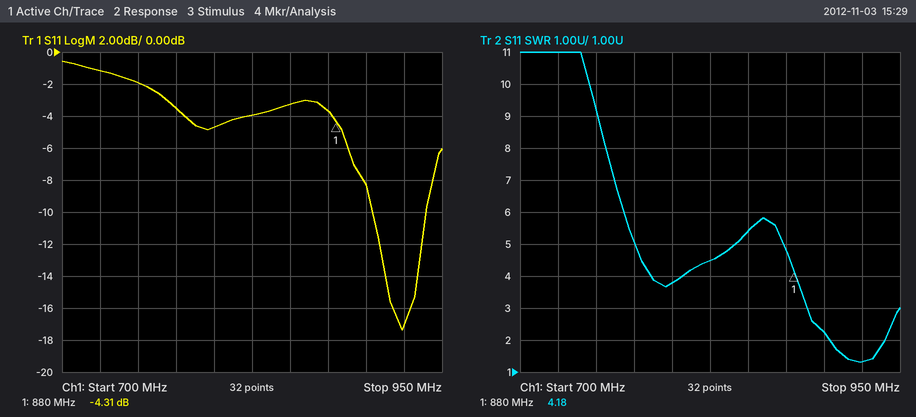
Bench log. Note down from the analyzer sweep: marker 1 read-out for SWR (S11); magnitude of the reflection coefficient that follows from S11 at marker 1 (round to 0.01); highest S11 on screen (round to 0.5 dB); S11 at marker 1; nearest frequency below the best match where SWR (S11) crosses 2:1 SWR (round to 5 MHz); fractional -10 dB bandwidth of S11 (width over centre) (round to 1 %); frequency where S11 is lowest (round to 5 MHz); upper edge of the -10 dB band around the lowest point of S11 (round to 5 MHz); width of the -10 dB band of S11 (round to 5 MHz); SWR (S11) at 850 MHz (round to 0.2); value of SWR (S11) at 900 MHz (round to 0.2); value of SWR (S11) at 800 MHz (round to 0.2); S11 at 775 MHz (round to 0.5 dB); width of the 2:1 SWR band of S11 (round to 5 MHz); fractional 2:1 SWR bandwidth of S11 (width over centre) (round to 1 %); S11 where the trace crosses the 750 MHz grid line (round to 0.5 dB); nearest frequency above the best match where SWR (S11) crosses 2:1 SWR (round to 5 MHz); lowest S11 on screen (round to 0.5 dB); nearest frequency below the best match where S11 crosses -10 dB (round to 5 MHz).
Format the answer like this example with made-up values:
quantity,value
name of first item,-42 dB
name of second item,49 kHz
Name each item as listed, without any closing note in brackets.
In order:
quantity,value
marker 1 read-out for SWR,4.18
magnitude of the reflection coefficient that follows from S11 at marker 1,0.61
highest S11 on screen,-0.5 dB
S11 at marker 1,-4.31 dB
nearest frequency below the best match where SWR (S11) crosses 2:1 SWR,905 MHz
fractional -10 dB bandwidth of S11 (width over centre),4 %
frequency where S11 is lowest,925 MHz
upper edge of the -10 dB band around the lowest point of S11,940 MHz
width of the -10 dB band of S11,35 MHz
SWR (S11) at 850 MHz,5.4
value of SWR (S11) at 900 MHz,2.2
value of SWR (S11) at 800 MHz,3.8
S11 at 775 MHz,-3.5 dB
width of the 2:1 SWR band of S11,35 MHz
fractional 2:1 SWR bandwidth of S11 (width over centre),4 %
S11 where the trace crosses the 750 MHz grid line,-2.0 dB
nearest frequency above the best match where SWR (S11) crosses 2:1 SWR,940 MHz
lowest S11 on screen,-17.5 dB
nearest frequency below the best match where S11 crosses -10 dB,905 MHz
